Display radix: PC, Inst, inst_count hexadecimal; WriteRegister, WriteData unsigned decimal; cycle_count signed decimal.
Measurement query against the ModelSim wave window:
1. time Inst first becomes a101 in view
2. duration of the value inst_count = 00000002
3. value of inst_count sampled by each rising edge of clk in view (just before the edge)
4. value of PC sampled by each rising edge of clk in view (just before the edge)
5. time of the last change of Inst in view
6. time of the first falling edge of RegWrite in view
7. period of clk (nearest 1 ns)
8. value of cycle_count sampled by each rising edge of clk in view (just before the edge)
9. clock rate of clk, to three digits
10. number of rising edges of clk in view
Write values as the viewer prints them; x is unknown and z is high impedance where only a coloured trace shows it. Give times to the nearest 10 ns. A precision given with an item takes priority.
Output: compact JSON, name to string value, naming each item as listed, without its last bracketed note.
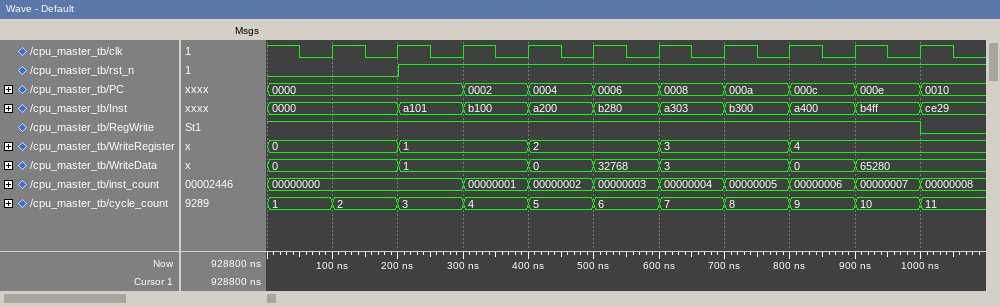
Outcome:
{"time Inst first becomes a101 in view": "200 ns", "duration of the value inst_count = 00000002": "100 ns", "value of inst_count sampled by each rising edge of clk in view": "00000000, 00000000, 00000000, 00000001, 00000002, 00000003, 00000004, 00000005, 00000006, 00000007", "value of PC sampled by each rising edge of clk in view": "0000, 0000, 0000, 0002, 0004, 0006, 0008, 000a, 000c, 000e", "time of the last change of Inst in view": "1000 ns", "time of the first falling edge of RegWrite in view": "1000 ns", "period of clk": "100 ns", "value of cycle_count sampled by each rising edge of clk in view": "1, 2, 3, 4, 5, 6, 7, 8, 9, 10", "clock rate of clk, to three digits": "10.0 MHz", "number of rising edges of clk in view": "10"}
